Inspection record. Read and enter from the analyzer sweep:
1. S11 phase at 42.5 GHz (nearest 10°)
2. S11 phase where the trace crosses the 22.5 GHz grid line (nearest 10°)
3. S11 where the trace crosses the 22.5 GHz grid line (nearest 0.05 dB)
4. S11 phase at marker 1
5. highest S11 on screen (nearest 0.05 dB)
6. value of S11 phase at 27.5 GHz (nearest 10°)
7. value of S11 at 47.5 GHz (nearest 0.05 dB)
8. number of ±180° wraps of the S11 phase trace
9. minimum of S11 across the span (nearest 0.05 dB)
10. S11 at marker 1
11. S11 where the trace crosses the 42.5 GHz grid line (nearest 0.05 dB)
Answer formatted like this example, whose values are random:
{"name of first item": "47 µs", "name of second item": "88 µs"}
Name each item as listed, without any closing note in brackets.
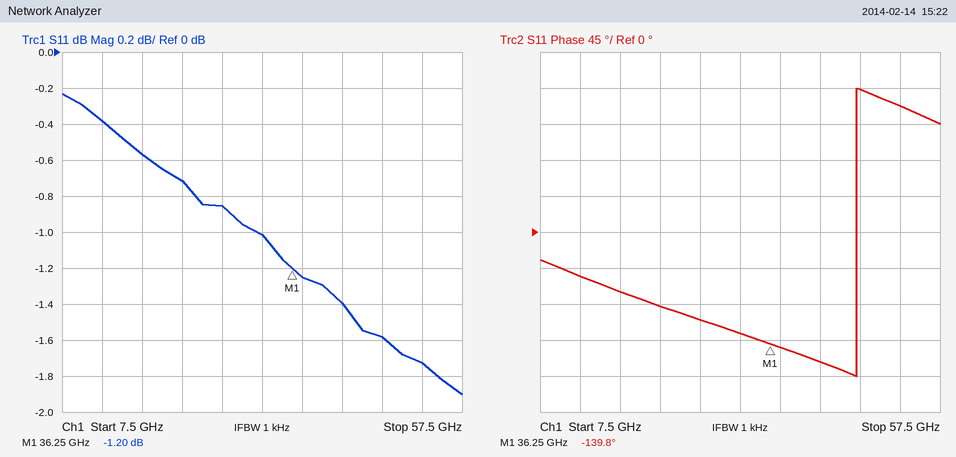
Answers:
{"S11 phase at 42.5 GHz": "-160°", "S11 phase where the trace crosses the 22.5 GHz grid line": "-90°", "S11 where the trace crosses the 22.5 GHz grid line": "-0.70 dB", "S11 phase at marker 1": "-139.8°", "highest S11 on screen": "-0.25 dB", "value of S11 phase at 27.5 GHz": "-110°", "value of S11 at 47.5 GHz": "-1.60 dB", "number of ±180° wraps of the S11 phase trace": "1", "minimum of S11 across the span": "-1.90 dB", "S11 at marker 1": "-1.20 dB", "S11 where the trace crosses the 42.5 GHz grid line": "-1.40 dB"}
